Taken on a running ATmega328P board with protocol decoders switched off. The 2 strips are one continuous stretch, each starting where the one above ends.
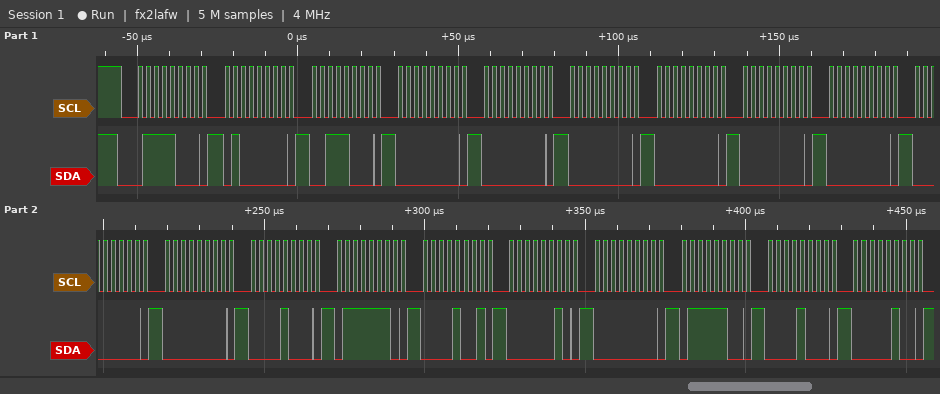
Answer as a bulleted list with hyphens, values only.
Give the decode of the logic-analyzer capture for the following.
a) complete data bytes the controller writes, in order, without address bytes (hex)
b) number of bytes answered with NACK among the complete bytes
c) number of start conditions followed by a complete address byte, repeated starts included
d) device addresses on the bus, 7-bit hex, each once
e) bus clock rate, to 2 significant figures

- 40 38 00 00 00 00 00 00 00 00 08 7E 09 02 00 7C 08 04
- 0
- 1
- 0x3C
- 400 kHz
